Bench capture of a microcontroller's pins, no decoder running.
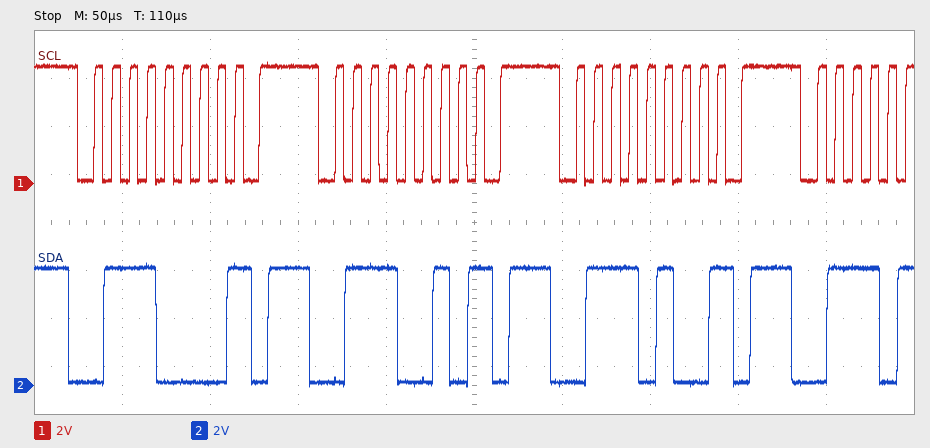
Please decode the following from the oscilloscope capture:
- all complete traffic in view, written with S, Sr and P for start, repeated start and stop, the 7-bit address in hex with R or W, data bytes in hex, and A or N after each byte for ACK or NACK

S 38W N P S 39W N P S 3AW N P
